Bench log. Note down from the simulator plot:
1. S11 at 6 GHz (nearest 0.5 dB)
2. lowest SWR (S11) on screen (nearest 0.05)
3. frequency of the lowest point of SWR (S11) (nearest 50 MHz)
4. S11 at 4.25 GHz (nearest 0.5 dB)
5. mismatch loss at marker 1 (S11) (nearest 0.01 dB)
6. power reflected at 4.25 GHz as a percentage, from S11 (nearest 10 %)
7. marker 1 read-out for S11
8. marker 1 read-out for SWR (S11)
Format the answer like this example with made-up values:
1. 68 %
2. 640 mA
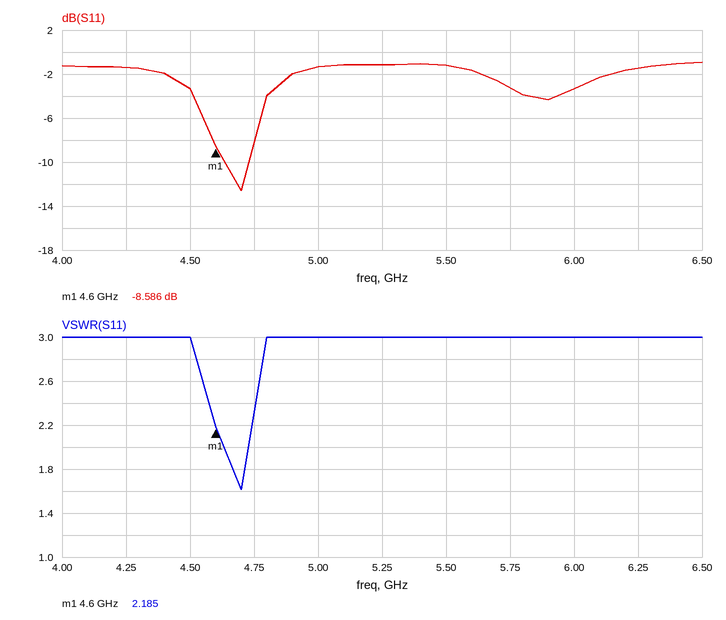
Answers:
1. -3.5 dB
2. 1.60
3. 4.70 GHz
4. -1.5 dB
5. 0.65 dB
6. 70 %
7. -8.586 dB
8. 2.185
